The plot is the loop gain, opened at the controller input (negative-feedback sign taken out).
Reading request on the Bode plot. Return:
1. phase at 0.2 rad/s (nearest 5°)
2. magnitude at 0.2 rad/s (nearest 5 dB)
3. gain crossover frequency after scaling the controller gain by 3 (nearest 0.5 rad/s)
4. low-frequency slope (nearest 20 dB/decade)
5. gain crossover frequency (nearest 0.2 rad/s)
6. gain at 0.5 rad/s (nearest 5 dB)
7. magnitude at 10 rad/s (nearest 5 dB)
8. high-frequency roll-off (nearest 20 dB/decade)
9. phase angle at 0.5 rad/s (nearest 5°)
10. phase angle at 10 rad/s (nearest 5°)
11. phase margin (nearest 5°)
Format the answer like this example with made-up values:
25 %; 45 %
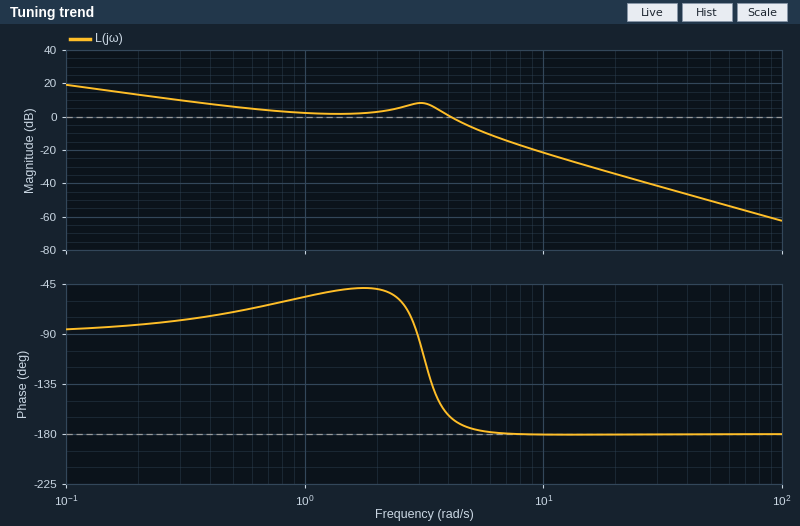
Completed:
-80°; 15 dB; 5.5 rad/s; -20 dB/decade; 4.0 rad/s; 5 dB; -20 dB; -40 dB/decade; -70°; -180°; 15°
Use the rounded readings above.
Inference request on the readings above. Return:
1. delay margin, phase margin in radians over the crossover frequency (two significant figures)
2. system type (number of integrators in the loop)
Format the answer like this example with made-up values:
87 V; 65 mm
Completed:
0.065 s; 1
